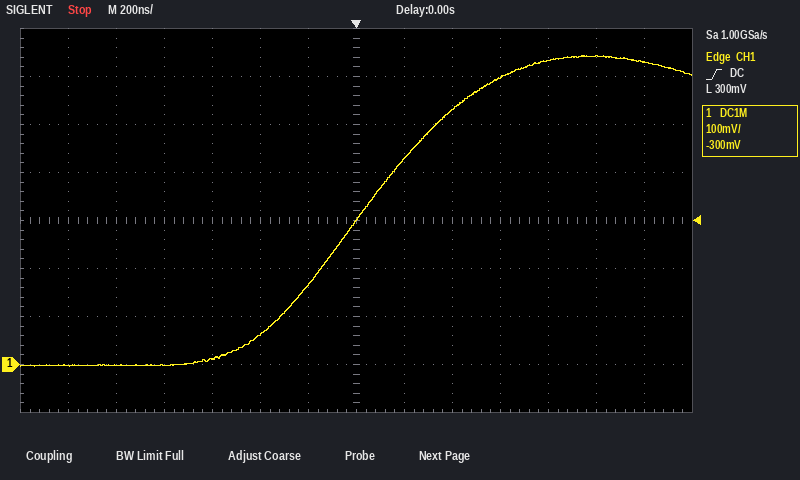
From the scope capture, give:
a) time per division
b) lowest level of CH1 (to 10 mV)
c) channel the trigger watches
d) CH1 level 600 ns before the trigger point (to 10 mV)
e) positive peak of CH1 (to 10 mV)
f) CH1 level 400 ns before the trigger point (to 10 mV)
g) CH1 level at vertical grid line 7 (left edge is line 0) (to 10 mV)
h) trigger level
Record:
200 ns
0 mV
CH1
10 mV
640 mV
60 mV
300 mV
300 mV
